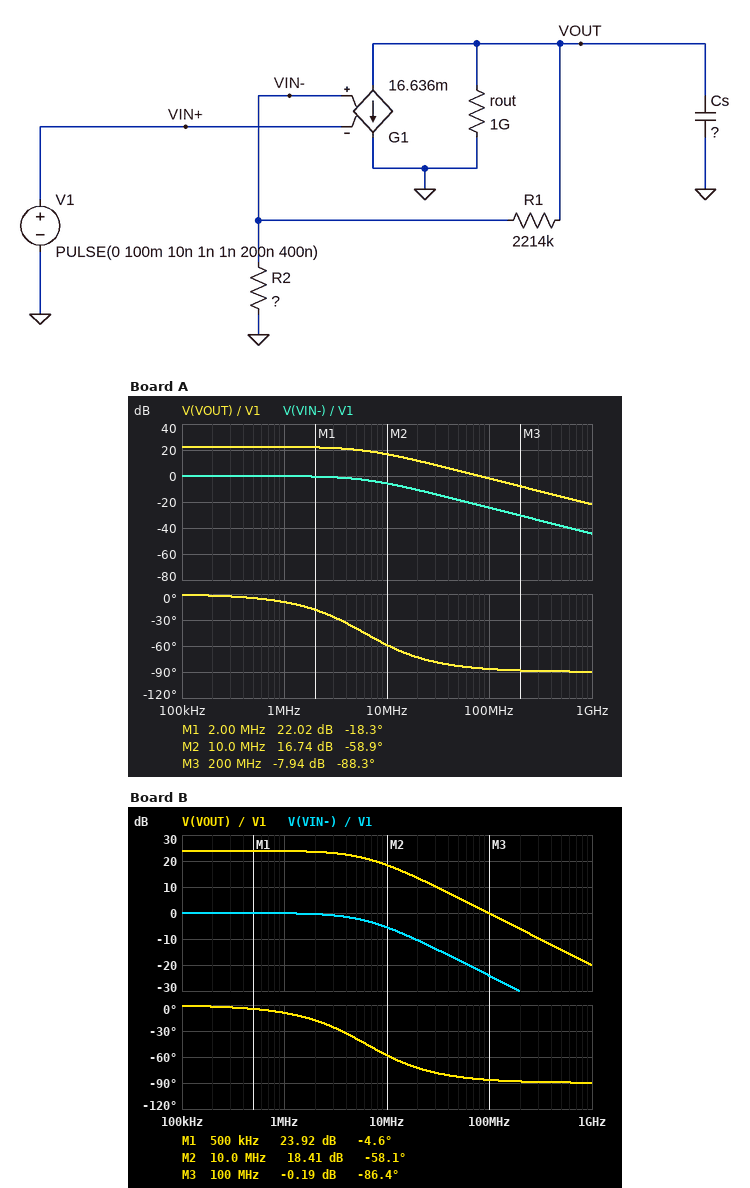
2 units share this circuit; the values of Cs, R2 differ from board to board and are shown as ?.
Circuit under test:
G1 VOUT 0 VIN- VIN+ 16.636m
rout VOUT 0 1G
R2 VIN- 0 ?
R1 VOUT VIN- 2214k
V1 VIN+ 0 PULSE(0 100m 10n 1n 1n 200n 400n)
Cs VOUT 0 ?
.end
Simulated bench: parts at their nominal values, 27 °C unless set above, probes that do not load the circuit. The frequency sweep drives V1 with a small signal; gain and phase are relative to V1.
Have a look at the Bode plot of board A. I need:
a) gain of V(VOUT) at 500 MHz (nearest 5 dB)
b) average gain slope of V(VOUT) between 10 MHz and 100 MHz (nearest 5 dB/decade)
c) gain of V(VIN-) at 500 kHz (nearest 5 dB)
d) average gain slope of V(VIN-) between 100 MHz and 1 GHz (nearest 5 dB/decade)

-15 dB
-20 dB/decade
0 dB
-20 dB/decade
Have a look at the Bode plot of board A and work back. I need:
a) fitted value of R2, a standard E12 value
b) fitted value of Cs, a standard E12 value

180 kΩ
33 pF
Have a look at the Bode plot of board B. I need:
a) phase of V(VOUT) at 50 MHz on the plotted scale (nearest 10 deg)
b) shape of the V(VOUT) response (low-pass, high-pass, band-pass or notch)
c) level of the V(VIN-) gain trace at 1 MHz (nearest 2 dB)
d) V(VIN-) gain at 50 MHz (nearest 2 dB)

-80 deg
low-pass
0 dB
-18 dB
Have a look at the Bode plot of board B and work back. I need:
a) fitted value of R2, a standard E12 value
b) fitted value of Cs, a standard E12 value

150 kΩ
27 pF
